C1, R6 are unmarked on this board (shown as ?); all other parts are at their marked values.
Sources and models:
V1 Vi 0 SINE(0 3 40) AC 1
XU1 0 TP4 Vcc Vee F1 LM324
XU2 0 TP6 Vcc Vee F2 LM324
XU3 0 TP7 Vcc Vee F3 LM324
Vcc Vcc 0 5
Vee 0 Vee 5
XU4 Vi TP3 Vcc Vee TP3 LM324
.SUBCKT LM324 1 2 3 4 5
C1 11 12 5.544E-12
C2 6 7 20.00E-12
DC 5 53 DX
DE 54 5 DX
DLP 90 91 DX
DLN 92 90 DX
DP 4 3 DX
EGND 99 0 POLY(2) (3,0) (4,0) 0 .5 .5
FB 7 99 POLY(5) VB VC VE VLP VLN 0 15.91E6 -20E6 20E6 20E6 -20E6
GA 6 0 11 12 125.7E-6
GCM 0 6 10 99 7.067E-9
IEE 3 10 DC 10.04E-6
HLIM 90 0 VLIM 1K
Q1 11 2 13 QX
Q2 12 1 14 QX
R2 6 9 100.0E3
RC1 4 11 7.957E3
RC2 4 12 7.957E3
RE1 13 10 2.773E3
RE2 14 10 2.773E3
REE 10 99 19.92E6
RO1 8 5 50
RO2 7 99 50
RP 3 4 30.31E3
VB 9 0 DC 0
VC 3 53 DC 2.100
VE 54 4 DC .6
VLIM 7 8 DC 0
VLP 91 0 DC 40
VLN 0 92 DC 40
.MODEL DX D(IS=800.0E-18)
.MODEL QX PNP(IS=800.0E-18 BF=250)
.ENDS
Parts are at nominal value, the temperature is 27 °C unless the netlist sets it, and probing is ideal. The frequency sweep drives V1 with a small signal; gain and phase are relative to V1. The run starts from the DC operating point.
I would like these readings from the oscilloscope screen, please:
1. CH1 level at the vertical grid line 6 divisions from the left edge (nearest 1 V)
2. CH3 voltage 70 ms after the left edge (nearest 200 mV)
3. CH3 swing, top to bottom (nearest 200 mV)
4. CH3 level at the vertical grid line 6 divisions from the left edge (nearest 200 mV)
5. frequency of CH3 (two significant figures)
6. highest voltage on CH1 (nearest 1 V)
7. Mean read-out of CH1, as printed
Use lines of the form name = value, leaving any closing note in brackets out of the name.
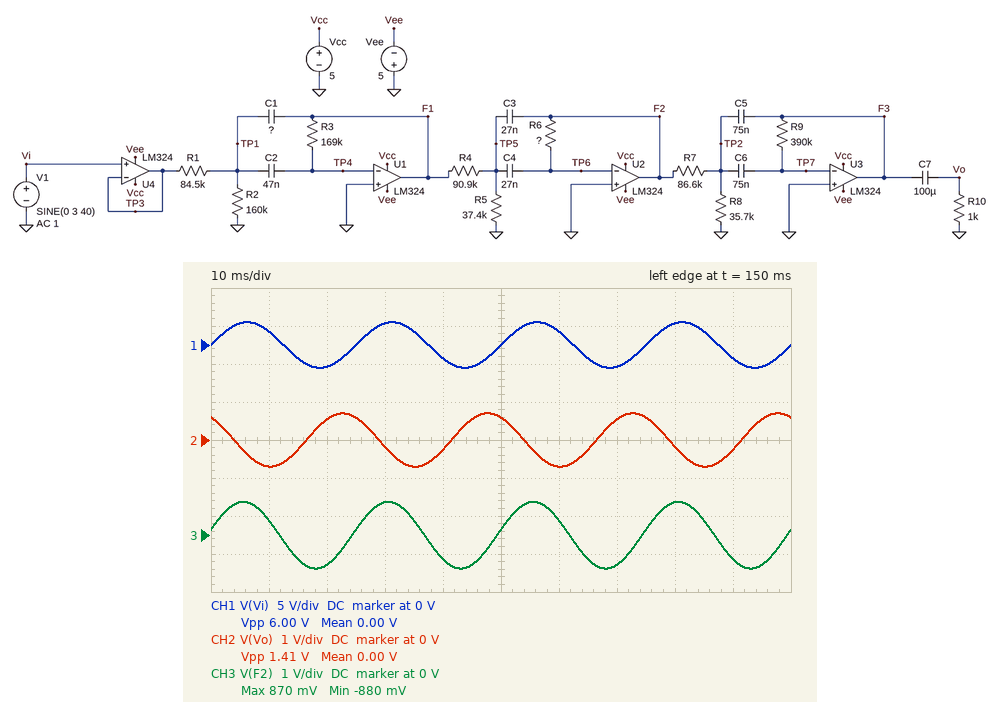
CH1 level at the vertical grid line 6 divisions from the left edge = 2 V
CH3 voltage 70 ms after the left edge = -800 mV
CH3 swing, top to bottom = 1.8 V
CH3 level at the vertical grid line 6 divisions from the left edge = 400 mV
frequency of CH3 = 40 Hz
highest voltage on CH1 = 3 V
Mean read-out of CH1, as printed = 0.00 V
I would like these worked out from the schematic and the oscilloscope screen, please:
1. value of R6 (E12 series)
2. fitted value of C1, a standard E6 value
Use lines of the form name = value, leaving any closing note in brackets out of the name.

value of R6 = 330 kΩ
fitted value of C1, a standard E6 value = 150 nF
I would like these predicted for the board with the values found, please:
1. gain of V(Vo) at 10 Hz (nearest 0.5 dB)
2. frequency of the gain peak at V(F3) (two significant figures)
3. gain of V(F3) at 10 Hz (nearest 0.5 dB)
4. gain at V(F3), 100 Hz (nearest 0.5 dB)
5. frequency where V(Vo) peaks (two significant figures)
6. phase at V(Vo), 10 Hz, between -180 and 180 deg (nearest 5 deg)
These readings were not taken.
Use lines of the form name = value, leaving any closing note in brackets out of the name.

gain of V(Vo) at 10 Hz = -29.0 dB
frequency of the gain peak at V(F3) = 23 Hz
gain of V(F3) at 10 Hz = -29.0 dB
gain at V(F3), 100 Hz = -30.5 dB
frequency where V(Vo) peaks = 23 Hz
phase at V(Vo), 10 Hz, between -180 and 180 deg = 35 deg
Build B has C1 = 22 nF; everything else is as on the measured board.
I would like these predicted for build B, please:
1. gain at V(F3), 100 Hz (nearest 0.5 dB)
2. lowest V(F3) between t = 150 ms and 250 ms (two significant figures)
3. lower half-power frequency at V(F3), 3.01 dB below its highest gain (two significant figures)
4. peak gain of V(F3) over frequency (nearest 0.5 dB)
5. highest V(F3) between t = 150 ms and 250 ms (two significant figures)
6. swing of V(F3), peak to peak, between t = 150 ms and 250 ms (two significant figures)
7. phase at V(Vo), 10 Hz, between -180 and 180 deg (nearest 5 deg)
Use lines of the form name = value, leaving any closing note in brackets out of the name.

gain at V(F3), 100 Hz = -13.5 dB
lowest V(F3) between t = 150 ms and 250 ms = -2.8 V
lower half-power frequency at V(F3), 3.01 dB below its highest gain = 30 Hz
peak gain of V(F3) over frequency = 1.0 dB
highest V(F3) between t = 150 ms and 250 ms = 2.8 V
swing of V(F3), peak to peak, between t = 150 ms and 250 ms = 5.6 V
phase at V(Vo), 10 Hz, between -180 and 180 deg = 65 deg
